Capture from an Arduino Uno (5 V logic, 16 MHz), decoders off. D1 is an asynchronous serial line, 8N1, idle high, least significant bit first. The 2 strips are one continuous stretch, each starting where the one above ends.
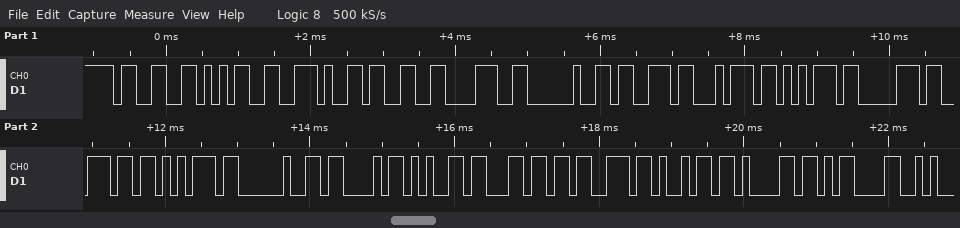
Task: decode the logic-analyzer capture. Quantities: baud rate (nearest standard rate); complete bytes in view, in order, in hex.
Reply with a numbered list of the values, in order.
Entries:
1. 9600 baud
2. 33 35 2E 33 38 20 73 74 75 70 6E 75 20 43 65 6C 73 69 61 0D
